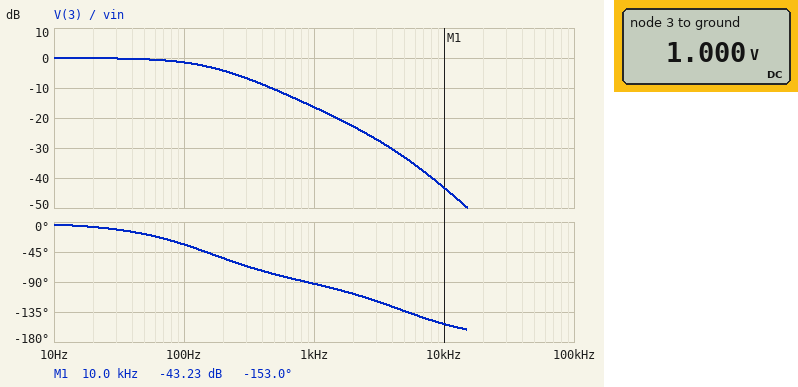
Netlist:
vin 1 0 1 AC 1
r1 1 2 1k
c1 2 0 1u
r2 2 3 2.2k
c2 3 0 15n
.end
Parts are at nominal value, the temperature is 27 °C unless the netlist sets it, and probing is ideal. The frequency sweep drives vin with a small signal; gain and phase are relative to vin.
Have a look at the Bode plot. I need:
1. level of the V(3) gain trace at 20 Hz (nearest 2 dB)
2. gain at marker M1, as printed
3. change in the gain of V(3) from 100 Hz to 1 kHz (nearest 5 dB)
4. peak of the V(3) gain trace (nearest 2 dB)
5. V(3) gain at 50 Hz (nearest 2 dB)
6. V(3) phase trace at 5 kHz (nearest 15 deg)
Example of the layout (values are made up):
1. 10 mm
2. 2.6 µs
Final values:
1. 0 dB
2. -43.23 dB
3. -15 dB
4. 0 dB
5. 0 dB
6. -135 deg
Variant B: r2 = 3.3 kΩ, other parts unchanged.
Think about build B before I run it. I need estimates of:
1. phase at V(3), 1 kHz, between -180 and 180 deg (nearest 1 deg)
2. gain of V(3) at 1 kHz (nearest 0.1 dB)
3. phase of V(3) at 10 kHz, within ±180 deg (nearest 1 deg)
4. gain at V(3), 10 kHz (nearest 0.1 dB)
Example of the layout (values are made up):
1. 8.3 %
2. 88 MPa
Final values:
1. -98 deg
2. -16.6 dB
3. -161 deg
4. -46.3 dB
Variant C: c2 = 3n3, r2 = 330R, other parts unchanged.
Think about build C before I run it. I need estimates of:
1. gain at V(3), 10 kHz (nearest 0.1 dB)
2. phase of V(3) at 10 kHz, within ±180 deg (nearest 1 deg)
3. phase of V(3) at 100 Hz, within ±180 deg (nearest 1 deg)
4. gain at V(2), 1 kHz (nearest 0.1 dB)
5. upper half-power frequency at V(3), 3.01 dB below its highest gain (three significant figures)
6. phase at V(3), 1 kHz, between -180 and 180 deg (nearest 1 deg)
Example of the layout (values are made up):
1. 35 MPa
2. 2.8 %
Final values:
1. -36.0 dB
2. -93 deg
3. -32 deg
4. -16.1 dB
5. 159 Hz
6. -81 deg
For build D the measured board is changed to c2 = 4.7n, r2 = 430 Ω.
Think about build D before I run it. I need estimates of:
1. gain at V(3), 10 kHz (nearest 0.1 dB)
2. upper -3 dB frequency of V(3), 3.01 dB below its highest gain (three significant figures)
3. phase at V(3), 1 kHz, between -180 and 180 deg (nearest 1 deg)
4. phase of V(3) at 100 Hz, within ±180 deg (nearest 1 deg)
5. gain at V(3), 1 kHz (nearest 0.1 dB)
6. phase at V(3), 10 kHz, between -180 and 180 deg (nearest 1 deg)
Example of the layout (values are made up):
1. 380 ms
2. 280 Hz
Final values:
1. -36.1 dB
2. 158 Hz
3. -82 deg
4. -32 deg
5. -16.1 dB
6. -96 deg
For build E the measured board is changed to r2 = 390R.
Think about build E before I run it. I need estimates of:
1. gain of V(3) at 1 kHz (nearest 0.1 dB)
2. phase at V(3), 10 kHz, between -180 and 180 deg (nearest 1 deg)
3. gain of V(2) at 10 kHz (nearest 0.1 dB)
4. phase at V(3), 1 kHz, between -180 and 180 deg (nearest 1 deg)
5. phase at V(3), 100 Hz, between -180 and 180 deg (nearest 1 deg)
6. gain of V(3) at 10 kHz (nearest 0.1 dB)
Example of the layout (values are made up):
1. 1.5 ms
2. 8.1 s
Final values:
1. -16.2 dB
2. -109 deg
3. -36.1 dB
4. -83 deg
5. -33 deg
6. -36.6 dB
